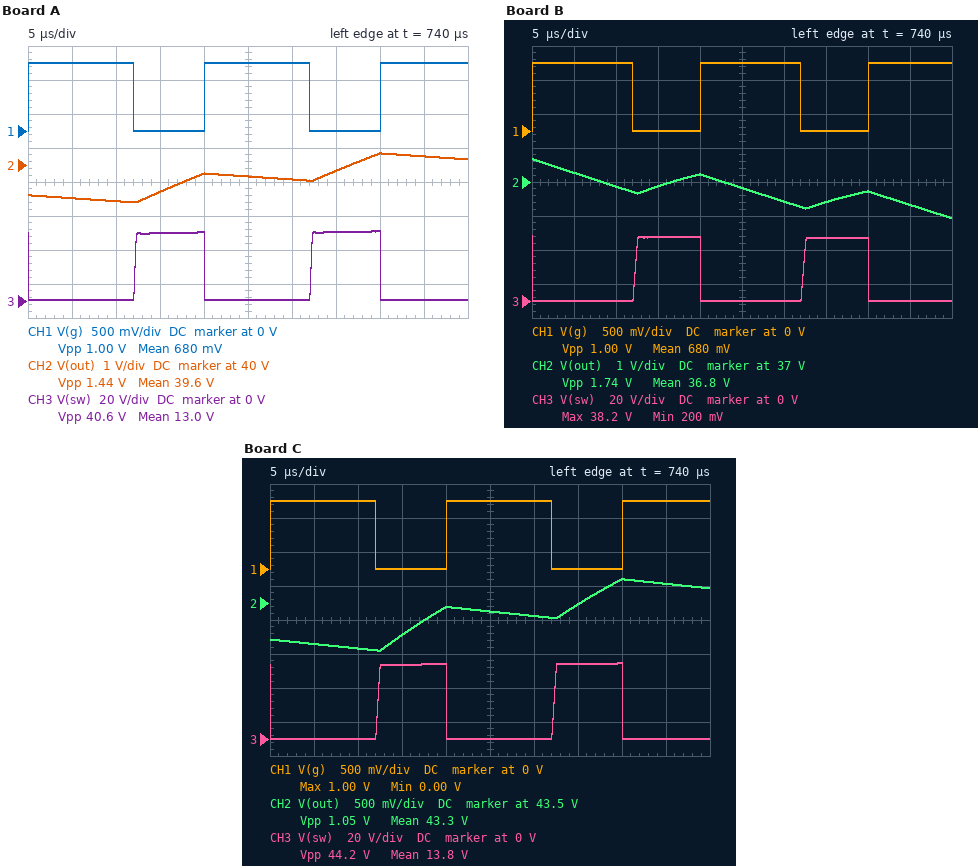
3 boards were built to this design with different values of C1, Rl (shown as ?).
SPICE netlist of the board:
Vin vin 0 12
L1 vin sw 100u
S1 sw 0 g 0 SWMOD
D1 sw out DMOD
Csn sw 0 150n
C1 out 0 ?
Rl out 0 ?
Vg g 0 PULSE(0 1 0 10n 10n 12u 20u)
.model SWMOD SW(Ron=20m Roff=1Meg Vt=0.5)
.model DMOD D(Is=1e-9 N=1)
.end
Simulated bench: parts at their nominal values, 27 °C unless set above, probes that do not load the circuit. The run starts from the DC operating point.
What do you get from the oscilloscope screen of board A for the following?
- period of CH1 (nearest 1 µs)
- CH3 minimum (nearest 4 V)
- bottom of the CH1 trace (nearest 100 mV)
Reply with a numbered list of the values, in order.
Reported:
1. 20 µs
2. 0 V
3. 0 V
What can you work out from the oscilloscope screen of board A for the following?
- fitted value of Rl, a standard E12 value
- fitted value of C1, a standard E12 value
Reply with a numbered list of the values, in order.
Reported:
1. 15 Ω
2. 150 µF
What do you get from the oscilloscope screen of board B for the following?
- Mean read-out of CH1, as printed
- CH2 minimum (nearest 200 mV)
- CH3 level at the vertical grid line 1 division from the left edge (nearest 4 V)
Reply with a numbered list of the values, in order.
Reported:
1. 680 mV
2. 36.0 V
3. 0 V
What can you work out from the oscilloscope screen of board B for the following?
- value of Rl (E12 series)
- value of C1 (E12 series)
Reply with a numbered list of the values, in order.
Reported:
1. 8.2 Ω
2. 56 µF
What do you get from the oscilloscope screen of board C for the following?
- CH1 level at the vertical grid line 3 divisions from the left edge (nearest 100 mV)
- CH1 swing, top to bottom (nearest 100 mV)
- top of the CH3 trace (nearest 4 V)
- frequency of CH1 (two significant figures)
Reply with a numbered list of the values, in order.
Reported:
1. 0 V
2. 1.0 V
3. 44 V
4. 50 kHz
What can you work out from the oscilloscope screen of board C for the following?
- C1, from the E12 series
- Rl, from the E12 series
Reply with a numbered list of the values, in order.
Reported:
1. 120 µF
2. 27 Ω
